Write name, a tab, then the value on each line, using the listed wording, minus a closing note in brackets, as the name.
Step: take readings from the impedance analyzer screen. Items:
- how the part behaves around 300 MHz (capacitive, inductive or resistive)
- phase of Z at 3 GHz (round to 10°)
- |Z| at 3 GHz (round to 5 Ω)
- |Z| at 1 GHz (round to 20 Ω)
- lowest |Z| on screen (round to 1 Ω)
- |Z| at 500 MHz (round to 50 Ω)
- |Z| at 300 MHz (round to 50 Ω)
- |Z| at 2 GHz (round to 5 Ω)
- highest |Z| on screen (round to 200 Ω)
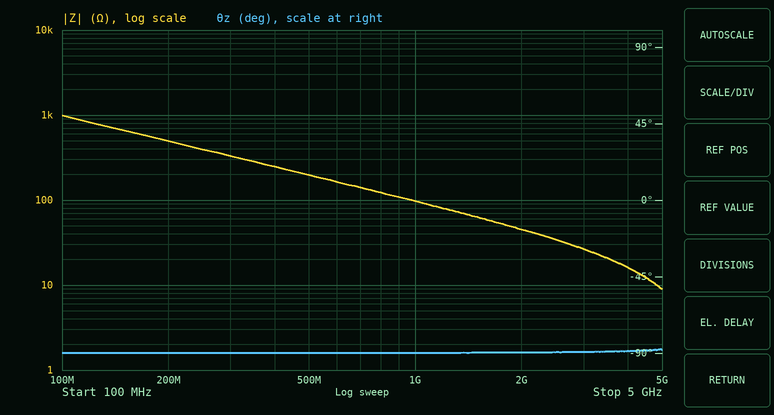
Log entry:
how the part behaves around 300 MHz	capacitive
phase of Z at 3 GHz	-90°
|Z| at 3 GHz	25 Ω
|Z| at 1 GHz	100 Ω
lowest |Z| on screen	9 Ω
|Z| at 500 MHz	200 Ω
|Z| at 300 MHz	350 Ω
|Z| at 2 GHz	45 Ω
highest |Z| on screen	1.0 kΩ
